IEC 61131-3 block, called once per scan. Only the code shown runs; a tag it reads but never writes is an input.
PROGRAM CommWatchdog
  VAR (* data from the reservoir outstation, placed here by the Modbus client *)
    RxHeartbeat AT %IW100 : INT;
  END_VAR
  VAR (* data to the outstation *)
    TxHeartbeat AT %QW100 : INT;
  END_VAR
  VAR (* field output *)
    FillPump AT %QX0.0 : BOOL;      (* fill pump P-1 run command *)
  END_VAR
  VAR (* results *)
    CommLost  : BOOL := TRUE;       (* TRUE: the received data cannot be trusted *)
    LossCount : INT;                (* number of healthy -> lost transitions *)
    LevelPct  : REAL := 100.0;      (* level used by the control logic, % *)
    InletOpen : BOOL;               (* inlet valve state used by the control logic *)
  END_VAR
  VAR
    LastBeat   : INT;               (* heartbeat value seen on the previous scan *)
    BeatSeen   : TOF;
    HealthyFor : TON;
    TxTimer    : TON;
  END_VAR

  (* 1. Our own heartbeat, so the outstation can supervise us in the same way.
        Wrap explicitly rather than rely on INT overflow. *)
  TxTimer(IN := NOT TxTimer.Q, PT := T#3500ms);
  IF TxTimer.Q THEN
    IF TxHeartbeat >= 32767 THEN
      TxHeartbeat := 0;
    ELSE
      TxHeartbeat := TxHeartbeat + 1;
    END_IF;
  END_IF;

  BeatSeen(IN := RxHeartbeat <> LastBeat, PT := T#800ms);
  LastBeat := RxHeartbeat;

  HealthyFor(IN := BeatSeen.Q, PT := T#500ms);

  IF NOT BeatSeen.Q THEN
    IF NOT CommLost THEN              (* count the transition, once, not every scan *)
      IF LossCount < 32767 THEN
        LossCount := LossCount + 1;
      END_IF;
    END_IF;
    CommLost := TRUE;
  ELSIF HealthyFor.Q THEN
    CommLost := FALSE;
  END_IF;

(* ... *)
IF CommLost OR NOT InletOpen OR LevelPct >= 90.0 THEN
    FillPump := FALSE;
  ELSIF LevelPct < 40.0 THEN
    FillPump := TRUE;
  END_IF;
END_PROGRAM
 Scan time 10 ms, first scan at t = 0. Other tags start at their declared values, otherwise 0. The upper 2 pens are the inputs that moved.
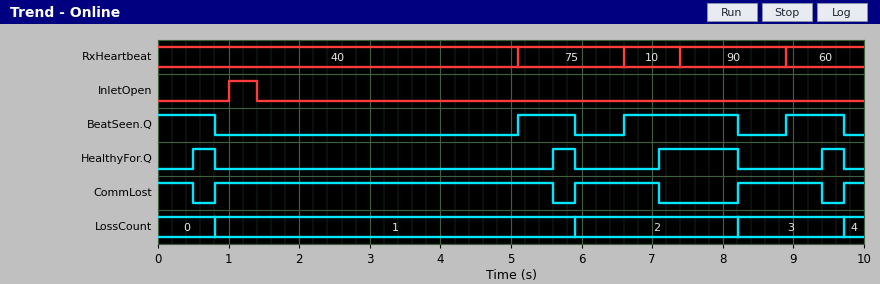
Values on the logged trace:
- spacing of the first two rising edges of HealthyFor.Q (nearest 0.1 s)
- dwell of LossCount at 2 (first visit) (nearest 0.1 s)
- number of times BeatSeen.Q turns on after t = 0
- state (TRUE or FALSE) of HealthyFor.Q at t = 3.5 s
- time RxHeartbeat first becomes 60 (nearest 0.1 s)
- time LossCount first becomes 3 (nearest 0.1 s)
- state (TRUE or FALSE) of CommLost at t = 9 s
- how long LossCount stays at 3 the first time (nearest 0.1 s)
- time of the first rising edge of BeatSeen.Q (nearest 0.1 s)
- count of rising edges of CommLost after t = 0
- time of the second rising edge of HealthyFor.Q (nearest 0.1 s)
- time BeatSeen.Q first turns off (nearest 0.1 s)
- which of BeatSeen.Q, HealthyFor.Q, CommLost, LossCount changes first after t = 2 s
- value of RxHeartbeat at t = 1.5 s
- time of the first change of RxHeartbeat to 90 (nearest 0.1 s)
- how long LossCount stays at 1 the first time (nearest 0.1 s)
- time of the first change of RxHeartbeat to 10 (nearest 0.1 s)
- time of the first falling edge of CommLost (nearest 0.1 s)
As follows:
5.1 s
2.3 s
3
FALSE
8.9 s
8.2 s
TRUE
1.5 s
5.1 s
4
5.6 s
0.8 s
BeatSeen.Q
40
7.4 s
5.1 s
6.6 s
0.5 s
